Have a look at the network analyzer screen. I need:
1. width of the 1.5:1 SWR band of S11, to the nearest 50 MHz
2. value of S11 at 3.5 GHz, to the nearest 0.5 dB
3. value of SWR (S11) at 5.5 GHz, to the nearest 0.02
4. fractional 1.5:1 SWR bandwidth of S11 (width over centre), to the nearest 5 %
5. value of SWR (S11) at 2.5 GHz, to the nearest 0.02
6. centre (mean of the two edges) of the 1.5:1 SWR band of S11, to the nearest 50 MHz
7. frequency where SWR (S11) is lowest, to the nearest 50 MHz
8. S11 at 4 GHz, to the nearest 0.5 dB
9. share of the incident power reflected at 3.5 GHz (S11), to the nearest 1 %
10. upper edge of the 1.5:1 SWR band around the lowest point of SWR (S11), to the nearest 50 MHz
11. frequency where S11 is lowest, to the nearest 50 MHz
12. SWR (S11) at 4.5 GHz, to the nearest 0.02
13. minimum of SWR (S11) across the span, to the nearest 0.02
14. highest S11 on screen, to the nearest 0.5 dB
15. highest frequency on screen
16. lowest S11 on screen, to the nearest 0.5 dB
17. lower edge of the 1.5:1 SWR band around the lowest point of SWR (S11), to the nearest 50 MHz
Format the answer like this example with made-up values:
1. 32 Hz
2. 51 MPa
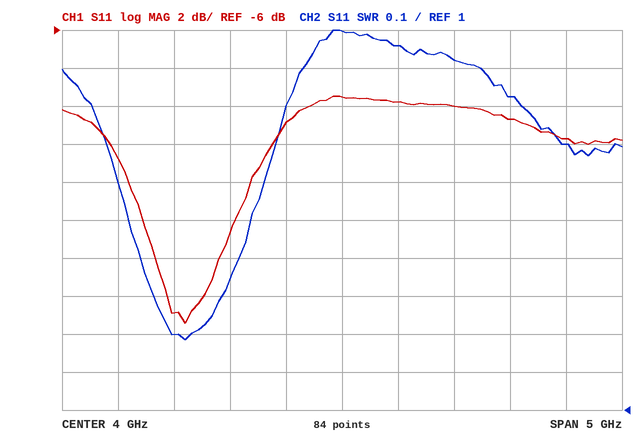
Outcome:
1. 1.10 GHz
2. -11.0 dB
3. 1.82
4. 40 %
5. 1.20
6. 2.65 GHz
7. 2.60 GHz
8. -9.5 dB
9. 8 %
10. 3.20 GHz
11. 2.60 GHz
12. 1.96
13. 1.18
14. -9.5 dB
15. 6.5 GHz
16. -21.5 dB
17. 2.10 GHz
